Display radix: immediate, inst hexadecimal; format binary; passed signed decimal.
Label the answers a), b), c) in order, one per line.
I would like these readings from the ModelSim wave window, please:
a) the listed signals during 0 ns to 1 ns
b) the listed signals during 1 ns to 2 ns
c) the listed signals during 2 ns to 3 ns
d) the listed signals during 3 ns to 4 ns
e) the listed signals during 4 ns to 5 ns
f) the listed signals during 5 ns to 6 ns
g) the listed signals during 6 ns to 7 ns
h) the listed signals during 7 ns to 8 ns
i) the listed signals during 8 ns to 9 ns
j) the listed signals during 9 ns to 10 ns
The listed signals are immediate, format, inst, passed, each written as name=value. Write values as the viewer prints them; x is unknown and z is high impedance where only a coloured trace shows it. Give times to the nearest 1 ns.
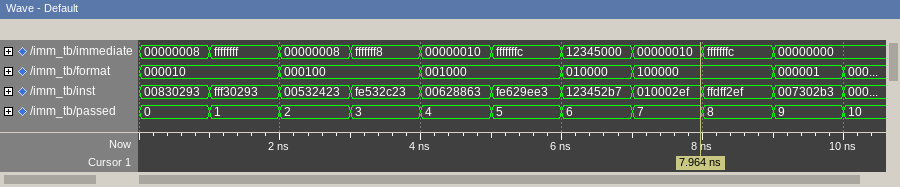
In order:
a) immediate=00000008, format=000010, inst=00830293, passed=0
b) immediate=ffffffff, format=000010, inst=fff30293, passed=1
c) immediate=00000008, format=000100, inst=00532423, passed=2
d) immediate=fffffff8, format=000100, inst=fe532c23, passed=3
e) immediate=00000010, format=001000, inst=00628863, passed=4
f) immediate=fffffffc, format=001000, inst=fe629ee3, passed=5
g) immediate=12345000, format=010000, inst=123452b7, passed=6
h) immediate=00000010, format=100000, inst=010002ef, passed=7
i) immediate=fffffffc, format=100000, inst=ffdff2ef, passed=8
j) immediate=00000000, format=000001, inst=007302b3, passed=9
